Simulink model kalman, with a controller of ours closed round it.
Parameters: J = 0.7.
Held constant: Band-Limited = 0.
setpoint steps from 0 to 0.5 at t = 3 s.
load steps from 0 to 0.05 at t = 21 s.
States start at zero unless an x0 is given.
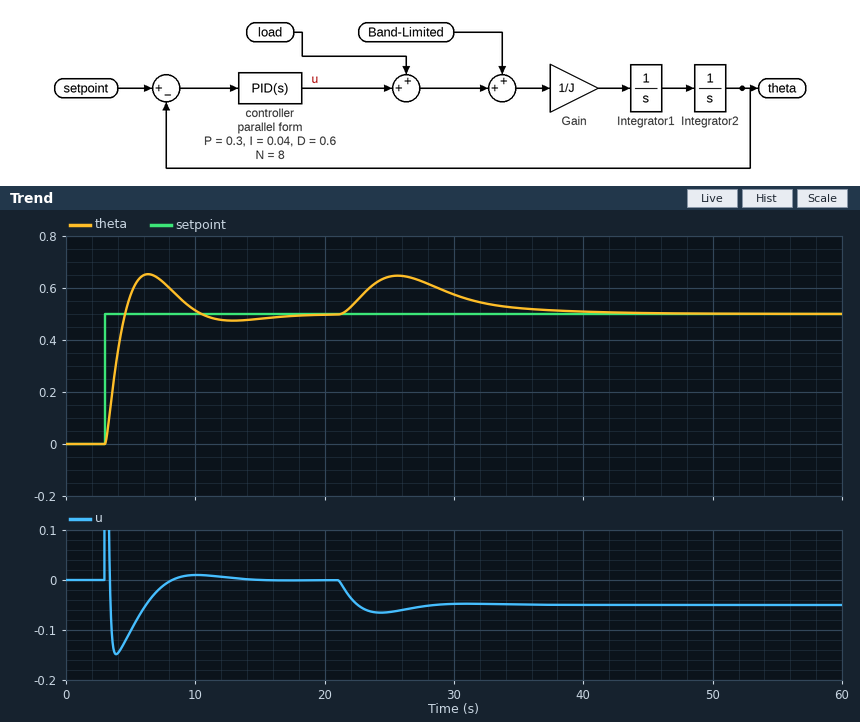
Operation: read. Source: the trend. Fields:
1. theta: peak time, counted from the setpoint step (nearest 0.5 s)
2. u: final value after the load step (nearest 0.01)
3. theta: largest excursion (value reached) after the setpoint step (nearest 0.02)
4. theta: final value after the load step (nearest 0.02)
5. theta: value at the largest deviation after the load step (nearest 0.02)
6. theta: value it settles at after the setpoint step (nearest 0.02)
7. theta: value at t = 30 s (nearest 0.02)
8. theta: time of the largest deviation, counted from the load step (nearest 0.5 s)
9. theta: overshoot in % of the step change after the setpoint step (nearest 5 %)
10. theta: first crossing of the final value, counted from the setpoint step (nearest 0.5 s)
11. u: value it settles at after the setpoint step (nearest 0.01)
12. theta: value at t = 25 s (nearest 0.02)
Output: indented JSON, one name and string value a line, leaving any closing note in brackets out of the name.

{
  "theta: peak time, counted from the setpoint step": "3.5 s",
  "u: final value after the load step": "-0.05",
  "theta: largest excursion (value reached) after the setpoint step": "0.66",
  "theta: final value after the load step": "0.50",
  "theta: value at the largest deviation after the load step": "0.64",
  "theta: value it settles at after the setpoint step": "0.50",
  "theta: value at t = 30 s": "0.58",
  "theta: time of the largest deviation, counted from the load step": "4.5 s",
  "theta: overshoot in % of the step change after the setpoint step": "30 %",
  "theta: first crossing of the final value, counted from the setpoint step": "1.5 s",
  "u: value it settles at after the setpoint step": "0.00",
  "theta: value at t = 25 s": "0.64"
}
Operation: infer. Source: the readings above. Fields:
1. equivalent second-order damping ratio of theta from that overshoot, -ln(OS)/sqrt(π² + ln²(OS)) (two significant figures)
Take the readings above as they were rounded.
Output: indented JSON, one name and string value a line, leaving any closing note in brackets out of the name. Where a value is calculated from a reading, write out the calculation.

{
  "equivalent second-order damping ratio of theta from that overshoot, -ln(OS)/sqrt(π² + ln²(OS))": "ln(0.3) = -1.204; 1.204 / sqrt(9.870 + 1.450) = 0.36"
}
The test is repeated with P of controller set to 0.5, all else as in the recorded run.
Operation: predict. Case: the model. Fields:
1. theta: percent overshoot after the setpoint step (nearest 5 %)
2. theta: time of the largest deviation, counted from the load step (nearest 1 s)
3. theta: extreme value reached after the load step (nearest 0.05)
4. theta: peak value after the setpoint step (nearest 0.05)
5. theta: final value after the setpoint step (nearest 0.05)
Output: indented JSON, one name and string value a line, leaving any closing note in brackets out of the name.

{
  "theta: percent overshoot after the setpoint step": "35 %",
  "theta: time of the largest deviation, counted from the load step": "4 s",
  "theta: extreme value reached after the load step": "0.60",
  "theta: peak value after the setpoint step": "0.70",
  "theta: final value after the setpoint step": "0.50"
}
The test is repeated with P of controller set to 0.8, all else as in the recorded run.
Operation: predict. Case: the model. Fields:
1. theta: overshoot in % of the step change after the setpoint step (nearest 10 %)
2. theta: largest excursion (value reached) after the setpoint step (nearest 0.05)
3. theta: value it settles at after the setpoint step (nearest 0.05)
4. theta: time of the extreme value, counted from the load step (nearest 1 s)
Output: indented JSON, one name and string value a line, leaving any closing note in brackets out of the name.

{
  "theta: overshoot in % of the step change after the setpoint step": "40 %",
  "theta: largest excursion (value reached) after the setpoint step": "0.70",
  "theta: value it settles at after the setpoint step": "0.50",
  "theta: time of the extreme value, counted from the load step": "3 s"
}
